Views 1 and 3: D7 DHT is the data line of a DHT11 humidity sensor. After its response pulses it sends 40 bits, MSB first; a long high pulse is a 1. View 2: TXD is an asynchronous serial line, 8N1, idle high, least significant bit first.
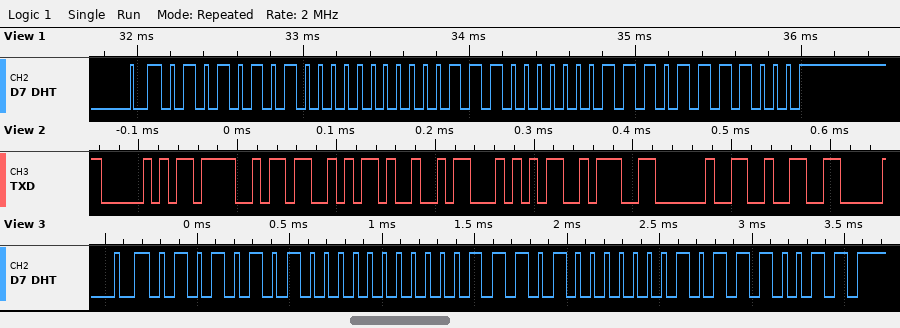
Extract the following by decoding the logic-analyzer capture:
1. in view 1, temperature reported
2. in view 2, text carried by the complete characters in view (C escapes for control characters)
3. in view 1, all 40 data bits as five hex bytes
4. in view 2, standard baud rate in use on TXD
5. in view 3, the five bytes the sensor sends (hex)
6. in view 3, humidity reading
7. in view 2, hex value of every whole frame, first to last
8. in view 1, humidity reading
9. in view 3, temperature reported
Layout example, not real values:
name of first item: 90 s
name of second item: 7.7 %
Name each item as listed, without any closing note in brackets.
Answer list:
in view 1, temperature reported: 28.7 °C
in view 2, text carried by the complete characters in view: "POSIT: 2"
in view 1, all 40 data bits as five hex bytes: 55 00 1C 07 78
in view 2, standard baud rate in use on TXD: 115200 baud
in view 3, the five bytes the sensor sends: 55 00 1D 01 73
in view 3, humidity reading: 85 %
in view 2, hex value of every whole frame, first to last: 50 4F 53 49 54 3A 20 32
in view 1, humidity reading: 85 %
in view 3, temperature reported: 29.1 °C
